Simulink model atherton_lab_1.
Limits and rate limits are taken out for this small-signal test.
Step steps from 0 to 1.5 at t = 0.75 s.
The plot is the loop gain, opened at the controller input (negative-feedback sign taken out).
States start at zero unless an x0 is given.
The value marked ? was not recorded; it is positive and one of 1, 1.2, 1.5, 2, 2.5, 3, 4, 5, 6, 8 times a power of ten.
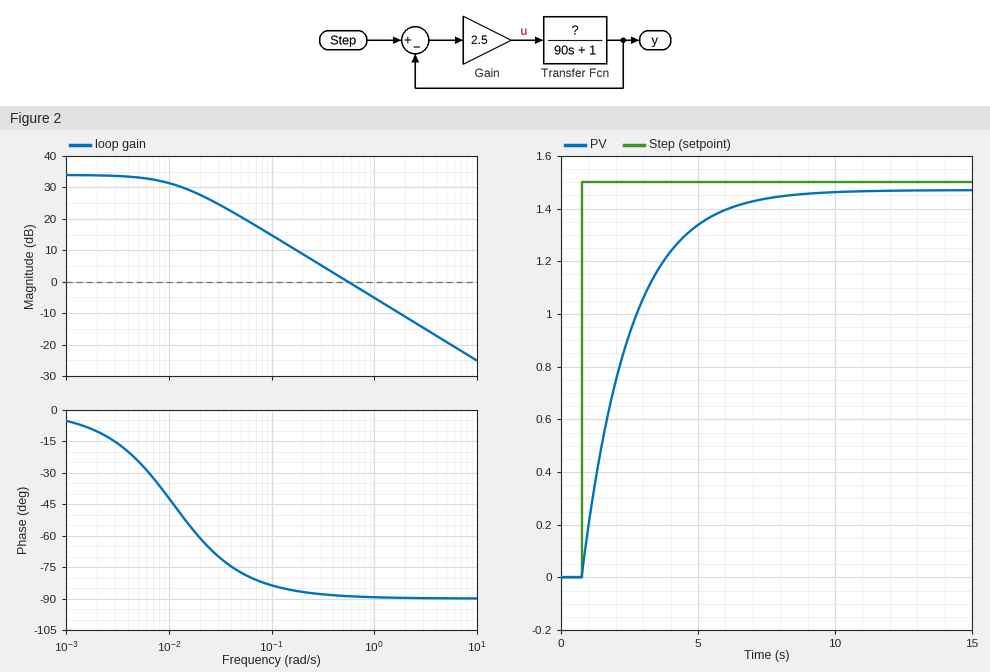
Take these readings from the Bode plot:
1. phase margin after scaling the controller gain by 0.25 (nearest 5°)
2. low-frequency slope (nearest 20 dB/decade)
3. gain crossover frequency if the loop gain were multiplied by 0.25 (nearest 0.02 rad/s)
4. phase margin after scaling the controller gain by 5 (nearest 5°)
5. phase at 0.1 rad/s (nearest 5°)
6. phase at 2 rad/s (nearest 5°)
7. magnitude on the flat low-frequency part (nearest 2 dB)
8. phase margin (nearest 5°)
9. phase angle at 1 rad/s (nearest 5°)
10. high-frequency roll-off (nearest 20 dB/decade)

95°
0 dB/decade
0.14 rad/s
90°
-85°
-90°
34 dB
90°
-90°
-20 dB/decade
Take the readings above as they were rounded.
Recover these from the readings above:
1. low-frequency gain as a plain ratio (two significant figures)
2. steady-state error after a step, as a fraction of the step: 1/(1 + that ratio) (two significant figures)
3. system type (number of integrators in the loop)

50
0.020
0
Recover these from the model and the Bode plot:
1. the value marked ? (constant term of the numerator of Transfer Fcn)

20
